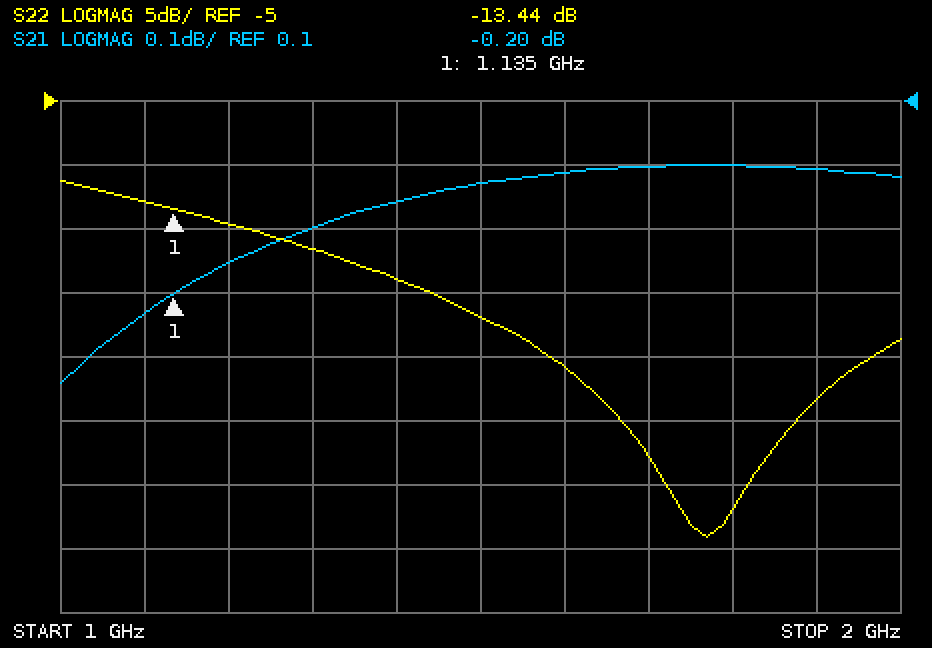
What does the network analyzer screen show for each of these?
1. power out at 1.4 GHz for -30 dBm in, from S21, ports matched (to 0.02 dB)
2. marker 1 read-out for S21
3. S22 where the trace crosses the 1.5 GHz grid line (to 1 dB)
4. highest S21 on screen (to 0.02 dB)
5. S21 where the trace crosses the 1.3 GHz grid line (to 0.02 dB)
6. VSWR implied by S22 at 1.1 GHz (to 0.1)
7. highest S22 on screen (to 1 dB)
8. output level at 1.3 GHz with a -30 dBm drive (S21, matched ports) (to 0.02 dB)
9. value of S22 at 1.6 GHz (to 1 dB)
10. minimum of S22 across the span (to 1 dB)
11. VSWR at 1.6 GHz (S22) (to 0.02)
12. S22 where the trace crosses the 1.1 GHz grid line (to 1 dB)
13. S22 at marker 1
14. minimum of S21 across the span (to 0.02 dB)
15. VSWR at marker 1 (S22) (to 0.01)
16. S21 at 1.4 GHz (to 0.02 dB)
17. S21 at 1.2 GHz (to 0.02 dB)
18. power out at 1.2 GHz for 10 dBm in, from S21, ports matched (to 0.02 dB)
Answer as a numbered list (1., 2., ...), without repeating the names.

1. -30.06 dBm
2. -0.20 dB
3. -22 dB
4. 0.00 dB
5. -0.10 dB
6. 1.6
7. -11 dB
8. -30.10 dBm
9. -26 dB
10. -39 dB
11. 1.10
12. -13 dB
13. -13.44 dB
14. -0.34 dB
15. 1.54
16. -0.06 dB
17. -0.16 dB
18. 9.84 dBm
